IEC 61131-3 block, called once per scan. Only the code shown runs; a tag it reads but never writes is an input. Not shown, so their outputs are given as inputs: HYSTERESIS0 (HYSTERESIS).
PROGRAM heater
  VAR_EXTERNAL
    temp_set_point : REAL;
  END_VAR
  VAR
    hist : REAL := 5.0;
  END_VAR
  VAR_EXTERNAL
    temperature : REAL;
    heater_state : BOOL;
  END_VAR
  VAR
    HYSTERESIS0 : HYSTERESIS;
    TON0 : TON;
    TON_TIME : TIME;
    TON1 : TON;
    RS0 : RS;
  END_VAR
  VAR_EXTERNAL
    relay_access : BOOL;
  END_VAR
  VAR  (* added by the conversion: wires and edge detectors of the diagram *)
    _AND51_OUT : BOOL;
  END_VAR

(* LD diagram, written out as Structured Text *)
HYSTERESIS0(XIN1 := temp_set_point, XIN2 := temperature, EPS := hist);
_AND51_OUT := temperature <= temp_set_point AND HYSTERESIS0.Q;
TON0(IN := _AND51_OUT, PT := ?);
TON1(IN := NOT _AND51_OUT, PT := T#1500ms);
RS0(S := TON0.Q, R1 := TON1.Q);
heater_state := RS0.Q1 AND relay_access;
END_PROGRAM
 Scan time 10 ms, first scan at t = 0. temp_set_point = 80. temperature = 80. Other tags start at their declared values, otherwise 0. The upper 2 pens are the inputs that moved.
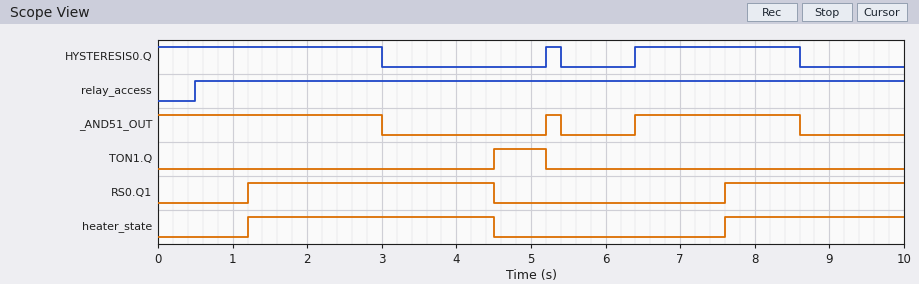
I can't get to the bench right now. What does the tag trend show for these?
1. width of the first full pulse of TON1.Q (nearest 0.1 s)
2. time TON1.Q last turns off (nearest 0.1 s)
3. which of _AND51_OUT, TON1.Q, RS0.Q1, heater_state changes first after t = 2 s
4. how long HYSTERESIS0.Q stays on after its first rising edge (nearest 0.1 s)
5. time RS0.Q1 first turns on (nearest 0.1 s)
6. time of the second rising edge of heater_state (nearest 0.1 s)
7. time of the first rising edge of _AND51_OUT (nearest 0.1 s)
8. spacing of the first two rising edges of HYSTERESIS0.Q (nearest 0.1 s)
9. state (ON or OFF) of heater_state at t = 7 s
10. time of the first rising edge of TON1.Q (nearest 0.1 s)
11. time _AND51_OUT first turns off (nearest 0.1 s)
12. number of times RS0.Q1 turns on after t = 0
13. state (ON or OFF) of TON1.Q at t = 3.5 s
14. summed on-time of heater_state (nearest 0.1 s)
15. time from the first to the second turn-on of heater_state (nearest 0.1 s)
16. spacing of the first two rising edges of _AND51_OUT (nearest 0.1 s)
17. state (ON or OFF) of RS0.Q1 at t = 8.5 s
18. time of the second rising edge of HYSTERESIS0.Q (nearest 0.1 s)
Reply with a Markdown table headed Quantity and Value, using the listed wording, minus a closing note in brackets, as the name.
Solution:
| Quantity | Value |
|---|---|
| width of the first full pulse of TON1.Q | 0.7 s |
| time TON1.Q last turns off | 5.2 s |
| which of _AND51_OUT, TON1.Q, RS0.Q1, heater_state changes first after t = 2 s | _AND51_OUT |
| how long HYSTERESIS0.Q stays on after its first rising edge | 0.2 s |
| time RS0.Q1 first turns on | 1.2 s |
| time of the second rising edge of heater_state | 7.6 s |
| time of the first rising edge of _AND51_OUT | 5.2 s |
| spacing of the first two rising edges of HYSTERESIS0.Q | 1.2 s |
| state (ON or OFF) of heater_state at t = 7 s | OFF |
| time of the first rising edge of TON1.Q | 4.5 s |
| time _AND51_OUT first turns off | 3.0 s |
| number of times RS0.Q1 turns on after t = 0 | 2 |
| state (ON or OFF) of TON1.Q at t = 3.5 s | OFF |
| summed on-time of heater_state | 5.7 s |
| time from the first to the second turn-on of heater_state | 6.4 s |
| spacing of the first two rising edges of _AND51_OUT | 1.2 s |
| state (ON or OFF) of RS0.Q1 at t = 8.5 s | ON |
| time of the second rising edge of HYSTERESIS0.Q | 6.4 s |
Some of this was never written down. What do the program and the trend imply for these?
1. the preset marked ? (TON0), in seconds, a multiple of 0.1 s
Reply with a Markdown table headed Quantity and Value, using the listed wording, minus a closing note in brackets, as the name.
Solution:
| Quantity | Value |
|---|---|
| the preset marked ? (TON0), in seconds, a multiple of 0.1 s | 1.2 s |
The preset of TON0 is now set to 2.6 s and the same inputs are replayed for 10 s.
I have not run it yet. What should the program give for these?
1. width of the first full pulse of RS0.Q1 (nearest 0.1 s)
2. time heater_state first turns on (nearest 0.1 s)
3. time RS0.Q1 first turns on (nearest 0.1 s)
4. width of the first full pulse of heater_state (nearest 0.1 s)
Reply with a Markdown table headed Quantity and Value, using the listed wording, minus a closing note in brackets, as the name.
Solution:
| Quantity | Value |
|---|---|
| width of the first full pulse of RS0.Q1 | 1.9 s |
| time heater_state first turns on | 2.6 s |
| time RS0.Q1 first turns on | 2.6 s |
| width of the first full pulse of heater_state | 1.9 s |
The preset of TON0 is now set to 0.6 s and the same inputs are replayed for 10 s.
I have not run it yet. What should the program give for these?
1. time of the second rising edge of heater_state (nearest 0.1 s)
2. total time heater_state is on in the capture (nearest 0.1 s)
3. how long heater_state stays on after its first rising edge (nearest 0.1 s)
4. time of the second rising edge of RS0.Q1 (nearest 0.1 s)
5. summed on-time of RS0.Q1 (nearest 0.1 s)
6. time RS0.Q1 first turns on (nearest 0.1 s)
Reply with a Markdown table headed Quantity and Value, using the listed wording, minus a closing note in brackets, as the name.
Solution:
| Quantity | Value |
|---|---|
| time of the second rising edge of heater_state | 7.0 s |
| total time heater_state is on in the capture | 6.9 s |
| how long heater_state stays on after its first rising edge | 3.9 s |
| time of the second rising edge of RS0.Q1 | 7.0 s |
| summed on-time of RS0.Q1 | 6.9 s |
| time RS0.Q1 first turns on | 0.6 s |
